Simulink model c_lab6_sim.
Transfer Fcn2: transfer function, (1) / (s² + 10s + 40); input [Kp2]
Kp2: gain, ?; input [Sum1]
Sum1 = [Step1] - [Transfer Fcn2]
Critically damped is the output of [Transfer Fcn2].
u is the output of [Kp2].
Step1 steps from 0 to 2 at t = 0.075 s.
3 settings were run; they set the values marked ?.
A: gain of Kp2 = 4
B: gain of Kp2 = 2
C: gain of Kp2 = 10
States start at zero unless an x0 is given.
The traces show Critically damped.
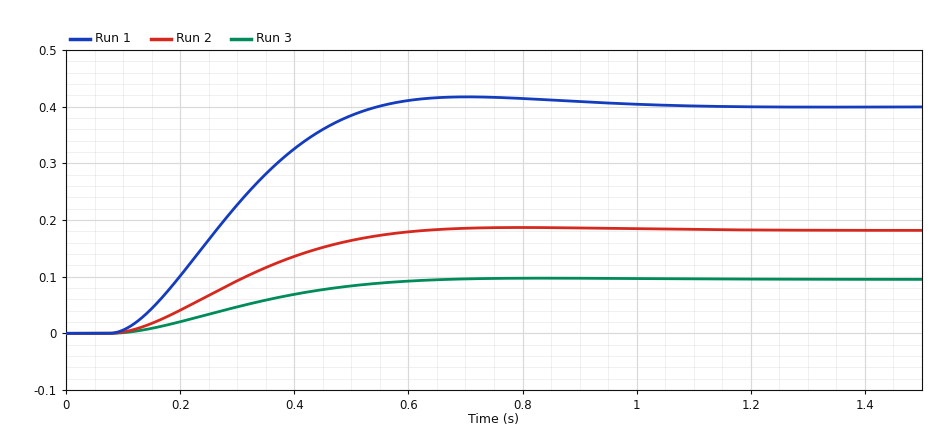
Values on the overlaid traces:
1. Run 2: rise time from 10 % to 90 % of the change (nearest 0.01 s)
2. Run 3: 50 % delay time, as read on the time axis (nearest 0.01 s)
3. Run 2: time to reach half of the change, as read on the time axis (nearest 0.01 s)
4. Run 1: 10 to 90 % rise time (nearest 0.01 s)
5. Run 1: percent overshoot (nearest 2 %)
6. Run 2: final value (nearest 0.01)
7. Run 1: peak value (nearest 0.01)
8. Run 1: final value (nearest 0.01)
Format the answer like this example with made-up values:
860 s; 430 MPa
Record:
0.35 s; 0.30 s; 0.30 s; 0.30 s; 4 %; 0.18; 0.42; 0.40
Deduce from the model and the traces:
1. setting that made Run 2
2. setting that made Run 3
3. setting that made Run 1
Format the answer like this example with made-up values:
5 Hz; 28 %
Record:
A; B; C
